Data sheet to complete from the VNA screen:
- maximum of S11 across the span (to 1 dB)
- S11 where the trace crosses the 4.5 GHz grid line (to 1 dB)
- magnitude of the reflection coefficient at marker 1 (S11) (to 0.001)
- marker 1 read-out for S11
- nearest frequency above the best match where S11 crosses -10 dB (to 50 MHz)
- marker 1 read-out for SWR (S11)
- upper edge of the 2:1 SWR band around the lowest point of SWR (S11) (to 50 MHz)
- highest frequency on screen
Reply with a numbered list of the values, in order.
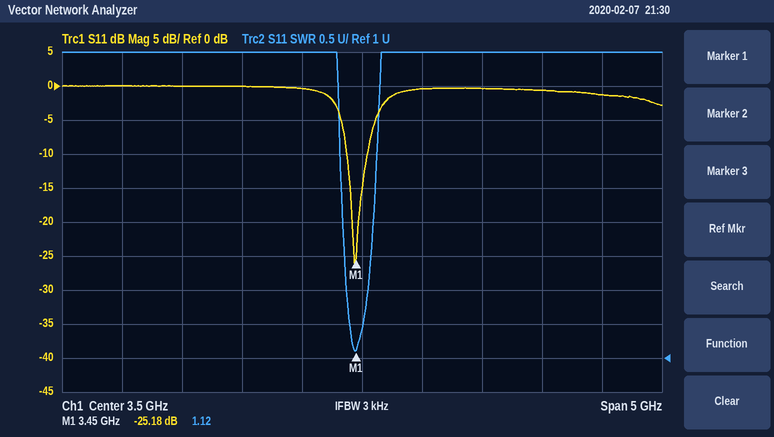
1. 0 dB
2. 0 dB
3. 0.055
4. -25.18 dB
5. 3.55 GHz
6. 1.12
7. 3.55 GHz
8. 6 GHz
